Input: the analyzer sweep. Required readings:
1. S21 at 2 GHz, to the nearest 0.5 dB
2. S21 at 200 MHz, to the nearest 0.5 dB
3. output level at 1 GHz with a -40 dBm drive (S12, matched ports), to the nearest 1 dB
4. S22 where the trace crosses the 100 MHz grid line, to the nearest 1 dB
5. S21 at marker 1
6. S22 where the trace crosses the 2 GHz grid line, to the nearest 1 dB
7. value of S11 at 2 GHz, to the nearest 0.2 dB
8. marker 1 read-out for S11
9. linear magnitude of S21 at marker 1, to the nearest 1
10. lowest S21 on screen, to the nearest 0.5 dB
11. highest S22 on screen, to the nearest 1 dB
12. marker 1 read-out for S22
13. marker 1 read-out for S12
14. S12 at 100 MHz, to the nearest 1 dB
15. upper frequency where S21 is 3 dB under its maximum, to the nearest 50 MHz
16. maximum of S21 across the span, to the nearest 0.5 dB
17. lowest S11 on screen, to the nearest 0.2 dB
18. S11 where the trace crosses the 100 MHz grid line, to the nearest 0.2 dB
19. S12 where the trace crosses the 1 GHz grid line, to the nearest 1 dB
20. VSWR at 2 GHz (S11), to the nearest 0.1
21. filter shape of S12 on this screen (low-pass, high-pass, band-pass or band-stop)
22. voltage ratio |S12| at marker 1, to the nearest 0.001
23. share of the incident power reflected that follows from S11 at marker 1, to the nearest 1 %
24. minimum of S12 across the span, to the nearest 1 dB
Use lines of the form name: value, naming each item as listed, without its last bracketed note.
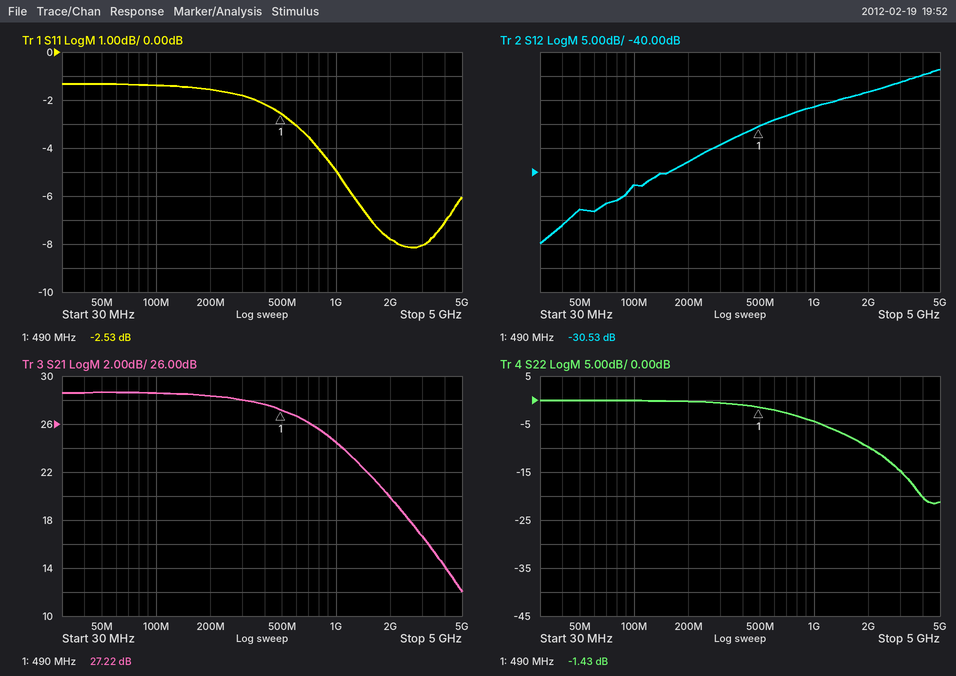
S21 at 2 GHz, to the nearest 0.5 dB: 20.0 dB
S21 at 200 MHz, to the nearest 0.5 dB: 28.5 dB
output level at 1 GHz with a -40 dBm drive (S12, matched ports), to the nearest 1 dB: -66 dBm
S22 where the trace crosses the 100 MHz grid line, to the nearest 1 dB: 0 dB
S21 at marker 1: 27.22 dB
S22 where the trace crosses the 2 GHz grid line, to the nearest 1 dB: -10 dB
value of S11 at 2 GHz, to the nearest 0.2 dB: -7.8 dB
marker 1 read-out for S11: -2.53 dB
linear magnitude of S21 at marker 1, to the nearest 1: 23
lowest S21 on screen, to the nearest 0.5 dB: 12.0 dB
highest S22 on screen, to the nearest 1 dB: 0 dB
marker 1 read-out for S22: -1.43 dB
marker 1 read-out for S12: -30.53 dB
S12 at 100 MHz, to the nearest 1 dB: -43 dB
upper frequency where S21 is 3 dB under its maximum, to the nearest 50 MHz: 800 MHz
maximum of S21 across the span, to the nearest 0.5 dB: 28.5 dB
lowest S11 on screen, to the nearest 0.2 dB: -8.2 dB
S11 where the trace crosses the 100 MHz grid line, to the nearest 0.2 dB: -1.4 dB
S12 where the trace crosses the 1 GHz grid line, to the nearest 1 dB: -26 dB
VSWR at 2 GHz (S11), to the nearest 0.1: 2.4
filter shape of S12 on this screen: high-pass
voltage ratio |S12| at marker 1, to the nearest 0.001: 0.030
share of the incident power reflected that follows from S11 at marker 1, to the nearest 1 %: 56 %
minimum of S12 across the span, to the nearest 1 dB: -55 dB
